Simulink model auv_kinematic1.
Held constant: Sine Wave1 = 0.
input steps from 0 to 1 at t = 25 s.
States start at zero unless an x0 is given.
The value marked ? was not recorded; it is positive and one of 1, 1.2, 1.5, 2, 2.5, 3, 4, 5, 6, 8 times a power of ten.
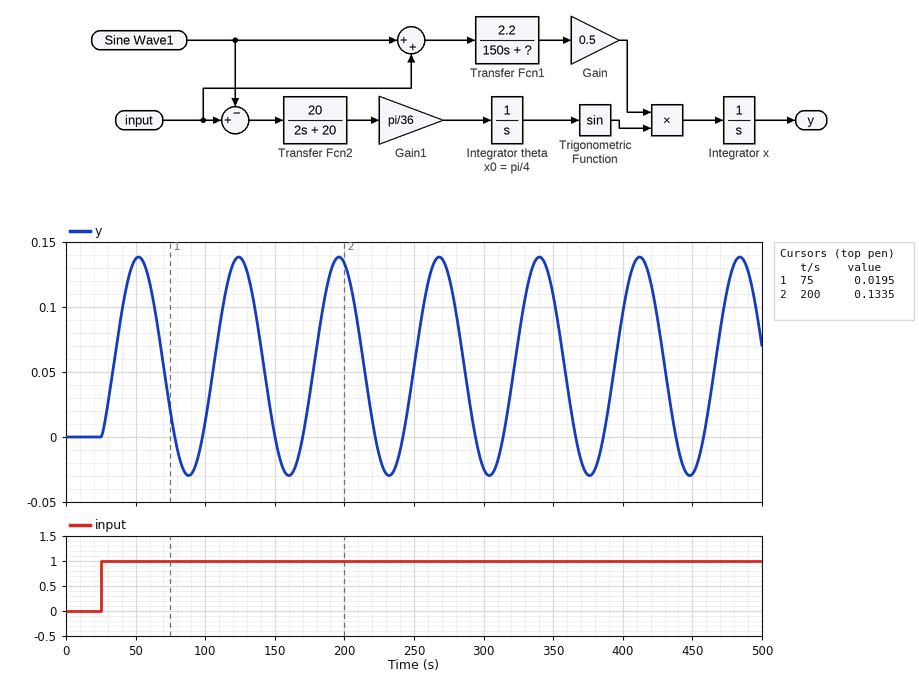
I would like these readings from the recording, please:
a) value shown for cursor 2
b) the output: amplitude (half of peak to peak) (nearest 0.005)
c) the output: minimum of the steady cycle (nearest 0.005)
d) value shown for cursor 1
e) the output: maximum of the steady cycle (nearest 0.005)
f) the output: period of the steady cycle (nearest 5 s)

0.1335
0.085
-0.030
0.0195
0.140
70 s
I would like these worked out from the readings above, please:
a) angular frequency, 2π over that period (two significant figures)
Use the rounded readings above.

0.090 rad/s
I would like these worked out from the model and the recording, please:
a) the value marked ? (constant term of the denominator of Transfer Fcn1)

150
